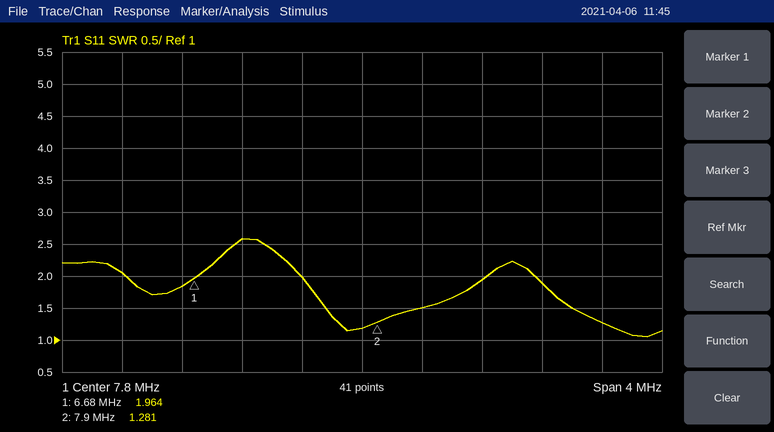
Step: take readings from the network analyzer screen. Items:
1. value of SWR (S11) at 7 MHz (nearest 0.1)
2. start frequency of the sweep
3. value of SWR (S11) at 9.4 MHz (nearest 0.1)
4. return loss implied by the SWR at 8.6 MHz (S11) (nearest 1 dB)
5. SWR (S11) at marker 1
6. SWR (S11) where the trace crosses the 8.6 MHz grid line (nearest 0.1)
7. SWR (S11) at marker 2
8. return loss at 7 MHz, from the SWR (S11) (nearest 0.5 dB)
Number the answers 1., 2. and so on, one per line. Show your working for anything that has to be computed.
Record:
1. 2.6
2. 5.8 MHz
3. 1.3
4. −20 log10((1.9 − 1)/(1.9 + 1)) ≈ 10 dB
5. 1.964
6. 1.9
7. 1.281
8. −20 log10((2.6 − 1)/(2.6 + 1)) ≈ 7.0 dB
